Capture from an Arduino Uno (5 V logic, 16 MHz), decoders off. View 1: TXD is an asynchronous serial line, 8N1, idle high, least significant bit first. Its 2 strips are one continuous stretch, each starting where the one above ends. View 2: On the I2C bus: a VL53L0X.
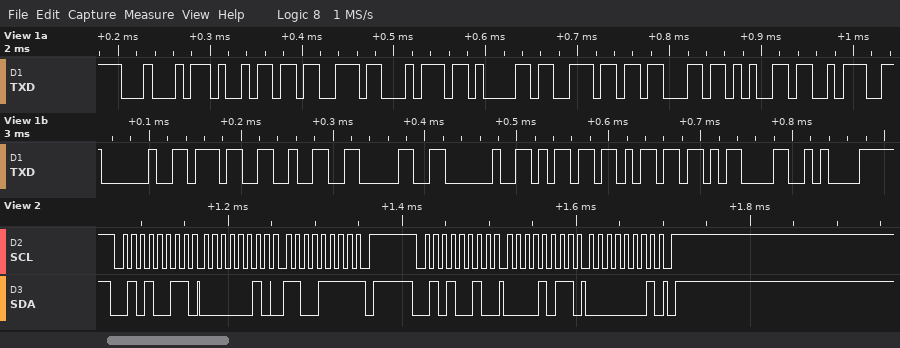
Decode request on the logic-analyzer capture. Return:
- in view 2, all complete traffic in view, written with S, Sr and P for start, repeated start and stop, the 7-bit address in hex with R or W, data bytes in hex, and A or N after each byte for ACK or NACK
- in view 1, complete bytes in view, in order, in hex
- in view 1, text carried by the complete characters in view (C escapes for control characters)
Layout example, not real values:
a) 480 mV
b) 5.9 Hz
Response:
a) S 29R A 02 A CF N P S 29W A 0B A 01 A P
b) 44 69 73 74 61 6E 63 65 3A 20 37 32 30 20 6D 6D 0D 0A
c) "Distance: 720 mm\r\n"
